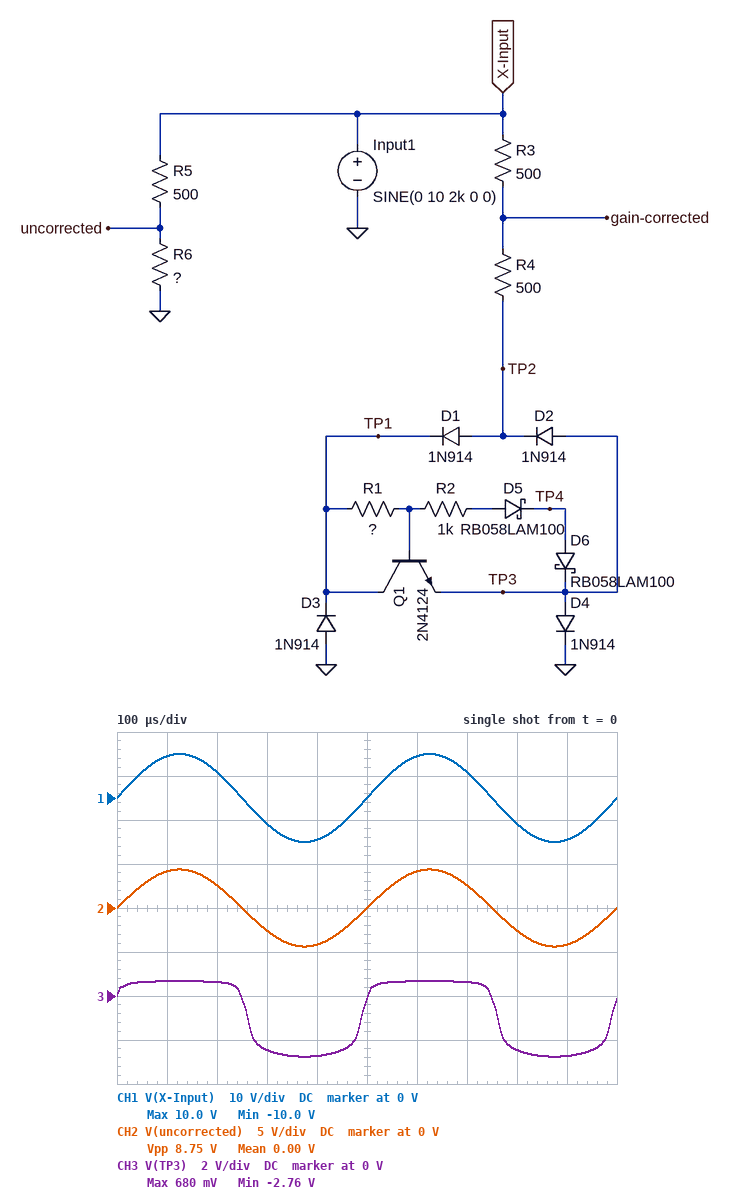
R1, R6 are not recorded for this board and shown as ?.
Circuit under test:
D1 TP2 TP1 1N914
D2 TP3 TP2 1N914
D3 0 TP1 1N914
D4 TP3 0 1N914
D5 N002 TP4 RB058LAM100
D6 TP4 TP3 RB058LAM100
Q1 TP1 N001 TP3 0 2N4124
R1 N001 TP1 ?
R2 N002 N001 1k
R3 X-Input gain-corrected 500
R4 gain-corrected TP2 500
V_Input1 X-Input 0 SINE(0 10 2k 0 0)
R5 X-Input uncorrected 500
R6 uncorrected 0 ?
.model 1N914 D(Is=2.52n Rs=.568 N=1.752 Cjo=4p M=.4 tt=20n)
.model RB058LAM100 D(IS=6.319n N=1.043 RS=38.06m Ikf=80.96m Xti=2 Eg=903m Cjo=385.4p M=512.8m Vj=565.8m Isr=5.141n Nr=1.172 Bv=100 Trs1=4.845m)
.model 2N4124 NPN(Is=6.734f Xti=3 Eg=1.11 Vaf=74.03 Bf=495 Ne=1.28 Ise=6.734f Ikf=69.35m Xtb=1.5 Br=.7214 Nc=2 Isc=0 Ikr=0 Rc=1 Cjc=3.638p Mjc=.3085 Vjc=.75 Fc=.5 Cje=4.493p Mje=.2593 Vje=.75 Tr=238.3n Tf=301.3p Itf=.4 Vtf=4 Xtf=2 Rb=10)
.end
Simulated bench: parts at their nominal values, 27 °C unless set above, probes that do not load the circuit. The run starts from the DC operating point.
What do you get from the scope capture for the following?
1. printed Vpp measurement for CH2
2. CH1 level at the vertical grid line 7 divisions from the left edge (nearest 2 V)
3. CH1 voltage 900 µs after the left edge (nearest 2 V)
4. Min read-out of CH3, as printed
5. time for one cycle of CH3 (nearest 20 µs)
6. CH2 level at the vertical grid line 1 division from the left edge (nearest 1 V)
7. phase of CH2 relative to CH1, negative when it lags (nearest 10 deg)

8.75 V
6 V
-10 V
-2.76 V
500 µs
4 V
0 deg
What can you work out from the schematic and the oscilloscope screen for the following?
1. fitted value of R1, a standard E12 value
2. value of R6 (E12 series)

6.8 kΩ
390 Ω
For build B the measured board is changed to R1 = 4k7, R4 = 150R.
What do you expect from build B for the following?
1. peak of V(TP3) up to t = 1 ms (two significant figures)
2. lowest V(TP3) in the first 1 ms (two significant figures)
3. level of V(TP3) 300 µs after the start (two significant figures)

700 mV
-2.5 V
-2.2 V
